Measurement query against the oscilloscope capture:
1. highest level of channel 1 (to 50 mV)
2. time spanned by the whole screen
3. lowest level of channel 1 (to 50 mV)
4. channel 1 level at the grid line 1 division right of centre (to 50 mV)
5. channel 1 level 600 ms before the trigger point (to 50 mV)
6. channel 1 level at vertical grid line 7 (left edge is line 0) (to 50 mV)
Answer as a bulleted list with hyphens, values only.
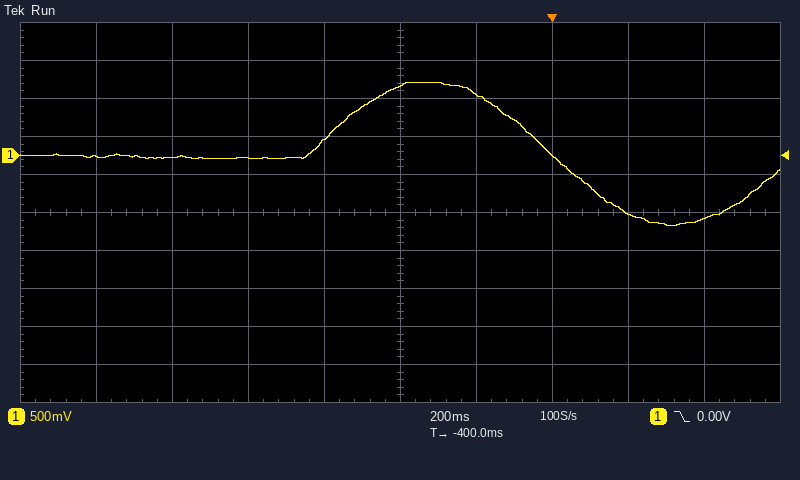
- 950 mV
- 2 s
- -900 mV
- 800 mV
- 200 mV
- 0 mV
